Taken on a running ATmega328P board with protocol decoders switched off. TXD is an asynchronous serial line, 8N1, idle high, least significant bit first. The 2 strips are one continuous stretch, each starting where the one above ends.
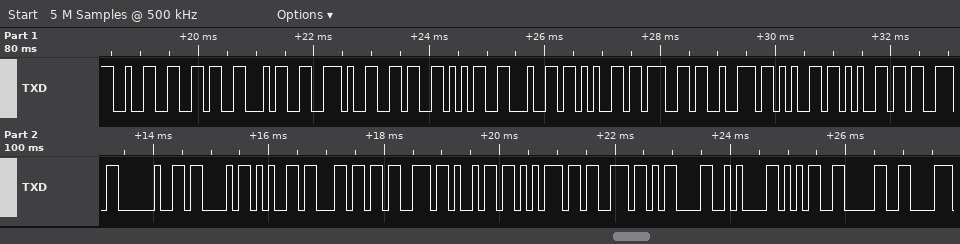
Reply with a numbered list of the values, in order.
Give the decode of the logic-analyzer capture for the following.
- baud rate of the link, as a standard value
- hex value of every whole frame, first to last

1. 9600 baud
2. 32 36 34 2E 36 35 64 65 67 72 65 65 73 20 43 65 6C 73 69 75 73 0D 0A 35 30
